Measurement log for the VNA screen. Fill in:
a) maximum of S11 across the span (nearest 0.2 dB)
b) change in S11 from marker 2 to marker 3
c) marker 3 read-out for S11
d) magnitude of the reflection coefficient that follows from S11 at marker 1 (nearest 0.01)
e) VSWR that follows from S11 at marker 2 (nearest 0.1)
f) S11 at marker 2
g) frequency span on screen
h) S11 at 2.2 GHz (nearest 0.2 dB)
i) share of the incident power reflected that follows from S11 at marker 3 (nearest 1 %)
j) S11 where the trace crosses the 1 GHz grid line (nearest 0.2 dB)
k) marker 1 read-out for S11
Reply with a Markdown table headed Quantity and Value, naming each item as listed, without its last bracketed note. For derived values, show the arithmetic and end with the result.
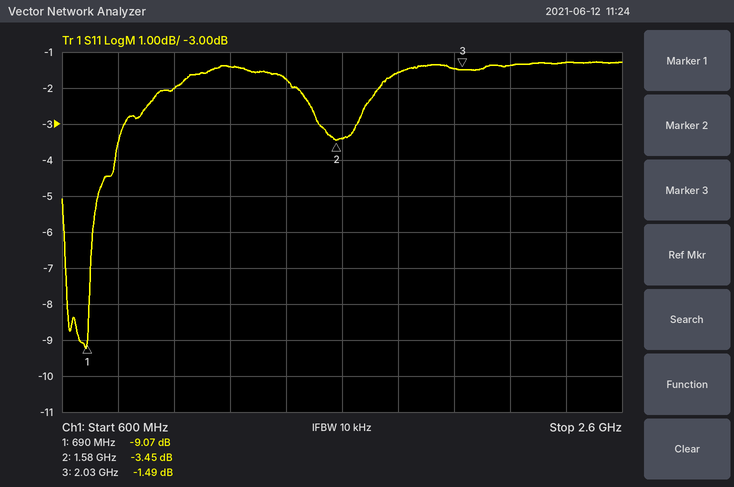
| Quantity | Value |
|---|---|
| maximum of S11 across the span | -1.2 dB |
| change in S11 from marker 2 to marker 3 | -1.49 − (-3.45) = 1.96 dB |
| marker 3 read-out for S11 | -1.49 dB |
| magnitude of the reflection coefficient that follows from S11 at marker 1 | 10^(-9.07/20) ≈ 0.35 |
| VSWR that follows from S11 at marker 2 | (1 + 0.6722)/(1 − 0.6722) ≈ 5.1 |
| S11 at marker 2 | -3.45 dB |
| frequency span on screen | 2 GHz |
| S11 at 2.2 GHz | -1.4 dB |
| share of the incident power reflected that follows from S11 at marker 3 | 10^(-1.49/10) ≈ 71 % |
| S11 where the trace crosses the 1 GHz grid line | -2.0 dB |
| marker 1 read-out for S11 | -9.07 dB |
